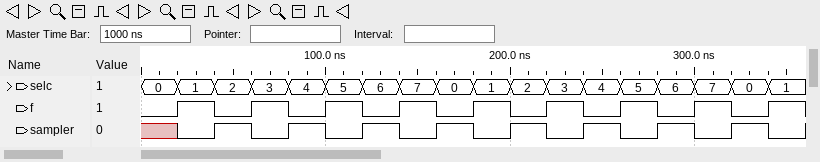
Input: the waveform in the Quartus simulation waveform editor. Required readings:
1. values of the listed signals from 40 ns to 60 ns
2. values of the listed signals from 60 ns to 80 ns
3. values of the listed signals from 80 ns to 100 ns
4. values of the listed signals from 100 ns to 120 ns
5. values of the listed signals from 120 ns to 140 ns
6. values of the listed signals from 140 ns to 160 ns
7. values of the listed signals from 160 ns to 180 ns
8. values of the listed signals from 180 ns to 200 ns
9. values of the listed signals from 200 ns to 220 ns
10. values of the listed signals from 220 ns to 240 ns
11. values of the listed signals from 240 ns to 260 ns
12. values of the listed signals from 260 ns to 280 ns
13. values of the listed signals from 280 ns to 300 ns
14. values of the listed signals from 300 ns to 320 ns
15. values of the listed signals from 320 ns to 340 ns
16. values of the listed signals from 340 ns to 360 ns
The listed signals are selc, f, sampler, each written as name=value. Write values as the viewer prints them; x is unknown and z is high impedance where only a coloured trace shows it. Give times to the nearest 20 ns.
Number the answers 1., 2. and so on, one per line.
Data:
1. selc=2, f=0, sampler=1
2. selc=3, f=1, sampler=0
3. selc=4, f=0, sampler=1
4. selc=5, f=1, sampler=0
5. selc=6, f=0, sampler=1
6. selc=7, f=1, sampler=0
7. selc=0, f=0, sampler=1
8. selc=1, f=1, sampler=0
9. selc=2, f=0, sampler=1
10. selc=3, f=1, sampler=0
11. selc=4, f=0, sampler=1
12. selc=5, f=1, sampler=0
13. selc=6, f=0, sampler=1
14. selc=7, f=1, sampler=0
15. selc=0, f=0, sampler=1
16. selc=1, f=1, sampler=0
